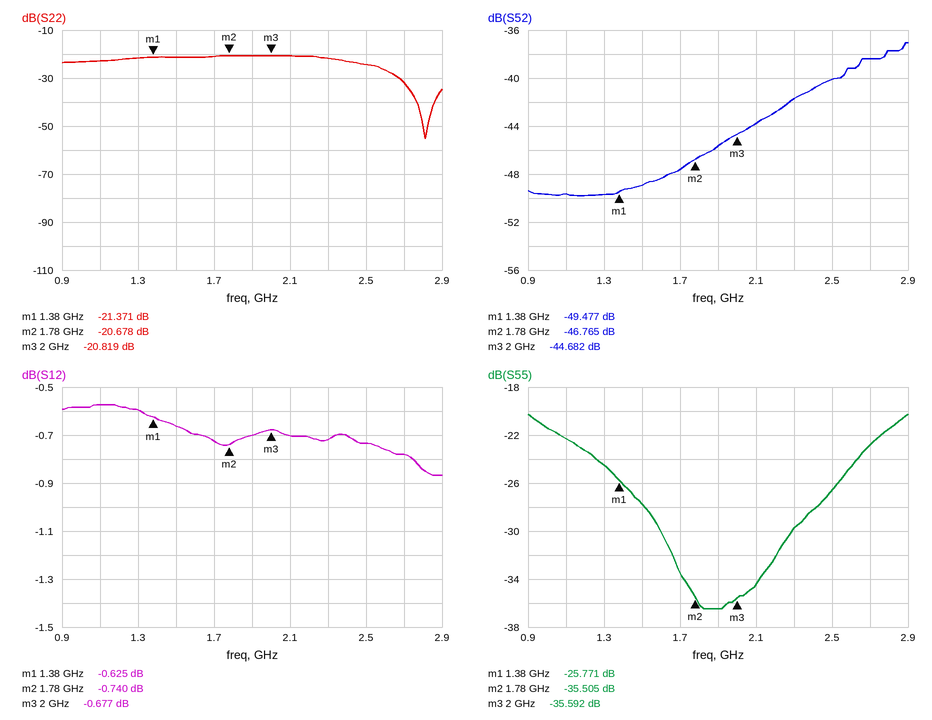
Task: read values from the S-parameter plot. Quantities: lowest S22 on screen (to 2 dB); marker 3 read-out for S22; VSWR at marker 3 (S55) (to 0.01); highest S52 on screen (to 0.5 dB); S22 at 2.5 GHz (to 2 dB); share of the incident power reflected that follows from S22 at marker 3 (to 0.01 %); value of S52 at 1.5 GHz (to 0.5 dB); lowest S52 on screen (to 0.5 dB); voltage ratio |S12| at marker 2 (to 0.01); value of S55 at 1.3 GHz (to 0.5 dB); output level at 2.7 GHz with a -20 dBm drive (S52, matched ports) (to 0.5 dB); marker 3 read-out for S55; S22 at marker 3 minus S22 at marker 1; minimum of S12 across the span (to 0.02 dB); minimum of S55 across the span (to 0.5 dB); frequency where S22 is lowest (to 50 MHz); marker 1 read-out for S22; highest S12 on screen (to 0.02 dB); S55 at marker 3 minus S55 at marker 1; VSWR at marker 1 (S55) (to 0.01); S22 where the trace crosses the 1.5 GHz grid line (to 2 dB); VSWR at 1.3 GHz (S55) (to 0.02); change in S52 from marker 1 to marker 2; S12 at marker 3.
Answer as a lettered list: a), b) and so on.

a) -56 dB
b) -20.819 dB
c) 1.03
d) -37.0 dB
e) -24 dB
f) 0.83 %
g) -49.0 dB
h) -50.0 dB
i) 0.92
j) -24.5 dB
k) -58.5 dBm
l) -35.592 dB
m) 0.552 dB
n) -0.86 dB
o) -36.5 dB
p) 2.80 GHz
q) -21.371 dB
r) -0.58 dB
s) -9.821 dB
t) 1.11
u) -22 dB
v) 1.12
w) 2.712 dB
x) -0.677 dB
